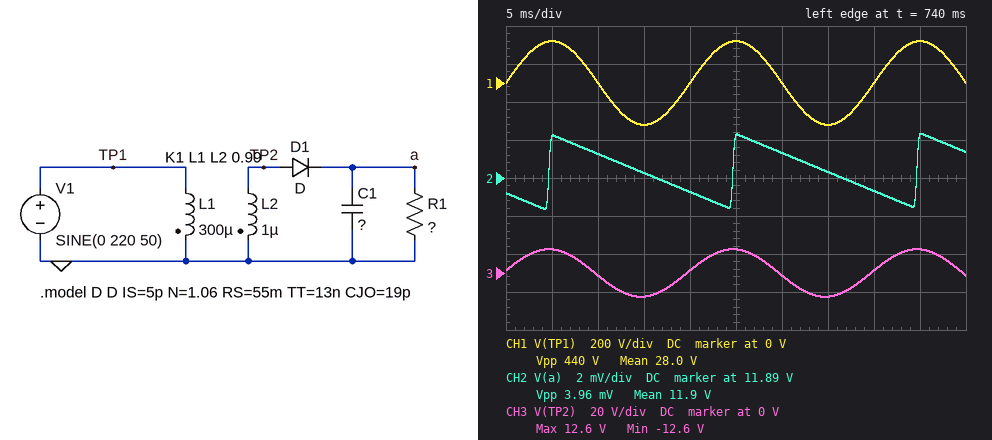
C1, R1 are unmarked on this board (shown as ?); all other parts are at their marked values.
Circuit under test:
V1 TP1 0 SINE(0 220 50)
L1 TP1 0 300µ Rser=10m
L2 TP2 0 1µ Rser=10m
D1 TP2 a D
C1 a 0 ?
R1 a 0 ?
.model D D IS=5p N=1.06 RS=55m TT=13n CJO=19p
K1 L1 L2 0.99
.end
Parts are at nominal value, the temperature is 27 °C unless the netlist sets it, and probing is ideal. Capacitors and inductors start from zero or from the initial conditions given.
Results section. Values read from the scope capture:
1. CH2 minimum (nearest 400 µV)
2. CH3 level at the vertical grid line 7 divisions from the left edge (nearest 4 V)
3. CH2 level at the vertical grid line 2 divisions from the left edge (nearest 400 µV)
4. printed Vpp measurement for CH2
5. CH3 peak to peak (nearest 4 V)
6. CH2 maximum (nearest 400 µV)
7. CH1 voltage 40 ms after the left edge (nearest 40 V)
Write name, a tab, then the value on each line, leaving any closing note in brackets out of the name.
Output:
CH2 minimum	11.8904 V
CH3 level at the vertical grid line 7 divisions from the left edge	-12 V
CH2 level at the vertical grid line 2 divisions from the left edge	11.8932 V
printed Vpp measurement for CH2	3.96 mV
CH3 peak to peak	24 V
CH2 maximum	11.8944 V
CH1 voltage 40 ms after the left edge	0 V
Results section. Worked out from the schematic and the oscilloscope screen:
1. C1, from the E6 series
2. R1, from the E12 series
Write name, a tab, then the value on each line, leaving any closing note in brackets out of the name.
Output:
C1, from the E6 series	2.2 mF
R1, from the E12 series	27 kΩ
